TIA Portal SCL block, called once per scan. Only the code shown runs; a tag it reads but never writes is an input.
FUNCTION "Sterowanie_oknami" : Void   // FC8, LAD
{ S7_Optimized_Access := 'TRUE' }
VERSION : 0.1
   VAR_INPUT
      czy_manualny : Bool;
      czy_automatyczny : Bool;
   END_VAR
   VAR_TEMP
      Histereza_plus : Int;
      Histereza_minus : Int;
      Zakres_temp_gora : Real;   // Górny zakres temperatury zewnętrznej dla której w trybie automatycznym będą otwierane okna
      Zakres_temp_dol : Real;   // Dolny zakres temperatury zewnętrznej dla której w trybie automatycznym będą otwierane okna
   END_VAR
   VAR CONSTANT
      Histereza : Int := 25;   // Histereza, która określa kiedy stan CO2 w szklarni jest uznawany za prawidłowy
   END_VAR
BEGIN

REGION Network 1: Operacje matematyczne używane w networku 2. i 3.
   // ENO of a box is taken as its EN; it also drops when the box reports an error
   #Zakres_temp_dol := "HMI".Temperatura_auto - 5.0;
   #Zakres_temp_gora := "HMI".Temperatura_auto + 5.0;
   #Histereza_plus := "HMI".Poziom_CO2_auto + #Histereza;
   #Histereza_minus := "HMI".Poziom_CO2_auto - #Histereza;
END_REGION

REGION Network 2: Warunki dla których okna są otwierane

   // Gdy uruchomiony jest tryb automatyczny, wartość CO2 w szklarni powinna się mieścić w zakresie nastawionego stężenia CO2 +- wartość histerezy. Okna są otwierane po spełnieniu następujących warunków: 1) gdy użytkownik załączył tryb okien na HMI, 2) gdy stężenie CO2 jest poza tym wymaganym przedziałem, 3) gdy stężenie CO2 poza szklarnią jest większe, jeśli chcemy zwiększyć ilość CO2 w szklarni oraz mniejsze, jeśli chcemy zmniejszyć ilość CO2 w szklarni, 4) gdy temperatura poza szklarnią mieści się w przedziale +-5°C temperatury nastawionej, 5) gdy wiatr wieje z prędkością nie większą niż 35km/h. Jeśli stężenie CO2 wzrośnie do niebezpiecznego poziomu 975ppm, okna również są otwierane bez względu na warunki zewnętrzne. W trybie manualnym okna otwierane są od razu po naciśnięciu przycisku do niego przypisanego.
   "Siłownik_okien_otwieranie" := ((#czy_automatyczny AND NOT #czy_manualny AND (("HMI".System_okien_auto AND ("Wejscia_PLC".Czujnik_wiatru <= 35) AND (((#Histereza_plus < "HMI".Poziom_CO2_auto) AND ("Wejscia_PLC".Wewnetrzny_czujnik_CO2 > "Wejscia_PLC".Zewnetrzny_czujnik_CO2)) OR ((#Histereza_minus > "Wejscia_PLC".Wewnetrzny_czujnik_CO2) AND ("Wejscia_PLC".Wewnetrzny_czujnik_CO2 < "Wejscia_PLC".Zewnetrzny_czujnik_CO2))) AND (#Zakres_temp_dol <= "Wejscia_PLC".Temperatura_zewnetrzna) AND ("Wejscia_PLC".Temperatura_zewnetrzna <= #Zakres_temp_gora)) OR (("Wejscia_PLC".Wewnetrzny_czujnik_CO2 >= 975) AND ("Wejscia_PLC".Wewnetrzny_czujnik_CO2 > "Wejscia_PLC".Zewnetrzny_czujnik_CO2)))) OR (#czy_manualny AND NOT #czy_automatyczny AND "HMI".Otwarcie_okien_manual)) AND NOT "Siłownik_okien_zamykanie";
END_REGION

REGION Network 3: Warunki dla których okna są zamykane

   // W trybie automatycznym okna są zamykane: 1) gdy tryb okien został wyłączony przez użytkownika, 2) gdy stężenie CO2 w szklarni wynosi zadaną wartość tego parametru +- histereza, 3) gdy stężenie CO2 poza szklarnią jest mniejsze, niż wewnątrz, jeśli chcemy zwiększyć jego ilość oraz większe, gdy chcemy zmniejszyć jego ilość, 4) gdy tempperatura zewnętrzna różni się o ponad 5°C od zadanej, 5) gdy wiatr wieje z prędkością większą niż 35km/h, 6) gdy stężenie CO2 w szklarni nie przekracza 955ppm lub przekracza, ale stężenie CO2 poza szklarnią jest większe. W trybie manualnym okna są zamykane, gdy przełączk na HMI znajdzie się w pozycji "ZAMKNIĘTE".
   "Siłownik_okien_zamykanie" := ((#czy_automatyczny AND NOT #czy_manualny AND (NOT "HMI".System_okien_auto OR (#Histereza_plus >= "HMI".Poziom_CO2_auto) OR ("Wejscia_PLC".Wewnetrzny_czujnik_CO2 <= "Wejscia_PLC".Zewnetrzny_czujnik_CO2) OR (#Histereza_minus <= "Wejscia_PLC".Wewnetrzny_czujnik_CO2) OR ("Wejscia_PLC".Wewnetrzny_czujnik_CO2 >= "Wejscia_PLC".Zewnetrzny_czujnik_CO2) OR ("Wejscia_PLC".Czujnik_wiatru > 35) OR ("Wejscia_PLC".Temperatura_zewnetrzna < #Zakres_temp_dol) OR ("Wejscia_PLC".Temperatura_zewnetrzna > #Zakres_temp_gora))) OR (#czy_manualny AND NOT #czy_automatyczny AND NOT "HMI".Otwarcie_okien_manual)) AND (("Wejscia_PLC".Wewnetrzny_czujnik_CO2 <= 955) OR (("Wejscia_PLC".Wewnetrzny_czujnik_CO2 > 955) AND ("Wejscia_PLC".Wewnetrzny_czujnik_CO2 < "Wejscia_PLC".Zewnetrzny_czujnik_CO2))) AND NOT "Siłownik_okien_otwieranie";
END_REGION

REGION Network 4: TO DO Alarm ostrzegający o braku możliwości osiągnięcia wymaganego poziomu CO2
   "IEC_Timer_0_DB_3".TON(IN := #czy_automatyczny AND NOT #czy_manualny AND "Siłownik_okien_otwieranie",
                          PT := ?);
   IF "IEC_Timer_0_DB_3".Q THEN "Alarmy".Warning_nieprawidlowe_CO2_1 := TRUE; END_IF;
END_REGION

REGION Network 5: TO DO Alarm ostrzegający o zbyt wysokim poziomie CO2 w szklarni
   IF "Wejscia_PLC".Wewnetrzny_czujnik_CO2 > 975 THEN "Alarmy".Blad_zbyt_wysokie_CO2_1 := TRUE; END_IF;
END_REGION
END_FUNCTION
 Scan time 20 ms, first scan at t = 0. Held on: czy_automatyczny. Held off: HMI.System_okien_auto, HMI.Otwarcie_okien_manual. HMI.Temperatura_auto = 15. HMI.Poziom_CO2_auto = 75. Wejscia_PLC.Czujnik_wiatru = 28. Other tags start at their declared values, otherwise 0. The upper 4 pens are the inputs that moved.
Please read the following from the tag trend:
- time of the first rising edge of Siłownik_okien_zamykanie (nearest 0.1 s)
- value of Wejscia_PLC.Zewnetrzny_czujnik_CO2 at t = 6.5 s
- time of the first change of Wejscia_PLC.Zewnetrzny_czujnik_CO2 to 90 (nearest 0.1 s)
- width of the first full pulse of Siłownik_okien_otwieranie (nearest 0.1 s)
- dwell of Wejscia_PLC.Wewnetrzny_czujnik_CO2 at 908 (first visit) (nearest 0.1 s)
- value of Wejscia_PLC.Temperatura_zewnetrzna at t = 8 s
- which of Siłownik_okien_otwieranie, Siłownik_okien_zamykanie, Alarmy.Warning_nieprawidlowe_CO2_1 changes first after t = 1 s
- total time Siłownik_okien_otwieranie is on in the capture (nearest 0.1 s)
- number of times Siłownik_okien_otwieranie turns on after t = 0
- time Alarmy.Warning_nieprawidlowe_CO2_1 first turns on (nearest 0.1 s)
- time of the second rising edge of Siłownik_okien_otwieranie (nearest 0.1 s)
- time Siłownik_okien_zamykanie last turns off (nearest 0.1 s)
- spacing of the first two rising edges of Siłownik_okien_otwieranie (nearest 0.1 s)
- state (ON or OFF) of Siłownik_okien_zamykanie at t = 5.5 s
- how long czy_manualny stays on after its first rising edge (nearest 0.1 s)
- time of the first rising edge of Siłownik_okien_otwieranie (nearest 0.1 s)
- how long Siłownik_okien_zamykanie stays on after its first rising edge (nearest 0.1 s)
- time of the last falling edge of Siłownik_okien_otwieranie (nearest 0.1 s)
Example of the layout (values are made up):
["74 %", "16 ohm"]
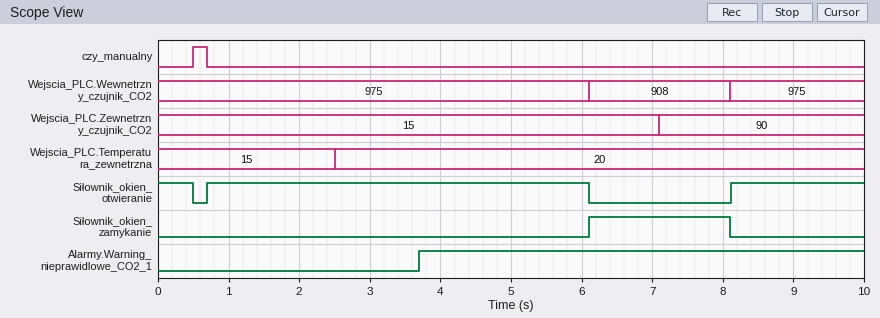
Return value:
["6.1 s", "15", "7.1 s", "5.4 s", "2.0 s", "20", "Alarmy.Warning_nieprawidlowe_CO2_1", "7.8 s", "2", "3.7 s", "8.1 s", "8.1 s", "7.4 s", "OFF", "0.2 s", "0.7 s", "2.0 s", "6.1 s"]
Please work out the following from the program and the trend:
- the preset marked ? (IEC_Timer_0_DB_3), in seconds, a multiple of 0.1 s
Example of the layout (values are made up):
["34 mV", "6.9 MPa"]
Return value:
["3.0 s"]
